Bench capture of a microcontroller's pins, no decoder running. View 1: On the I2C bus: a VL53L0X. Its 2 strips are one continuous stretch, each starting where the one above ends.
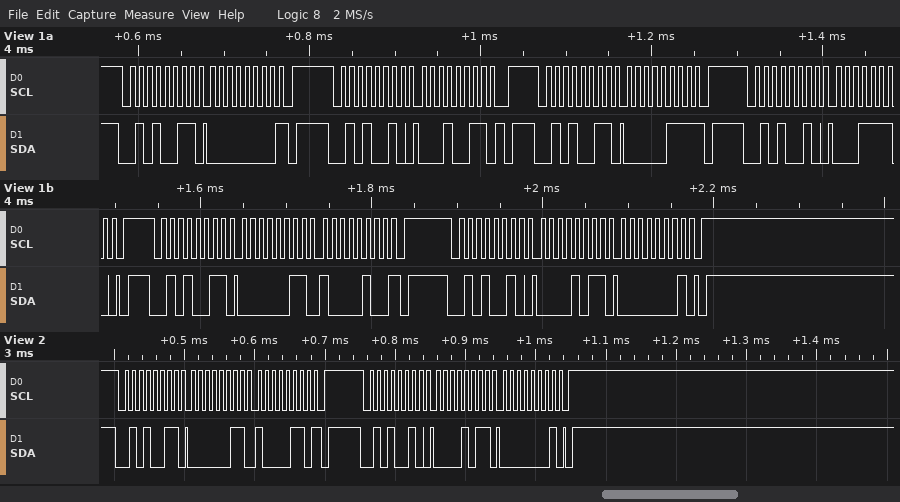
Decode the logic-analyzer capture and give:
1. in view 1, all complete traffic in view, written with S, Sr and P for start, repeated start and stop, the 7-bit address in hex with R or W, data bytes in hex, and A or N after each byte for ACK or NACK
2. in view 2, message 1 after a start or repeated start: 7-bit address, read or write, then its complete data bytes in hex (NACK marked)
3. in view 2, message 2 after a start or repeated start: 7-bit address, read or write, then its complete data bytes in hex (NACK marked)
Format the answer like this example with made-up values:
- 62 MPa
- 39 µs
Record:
- S 29R A 00 N P S 29W A 13 A P S 29R A 07 N P S 29W A 1E A P S 29R A 03 A 84 N P S 29W A 0B A 01 A P
- 0x29 read: 03 86 NACK
- 0x29 write: 0B 01
